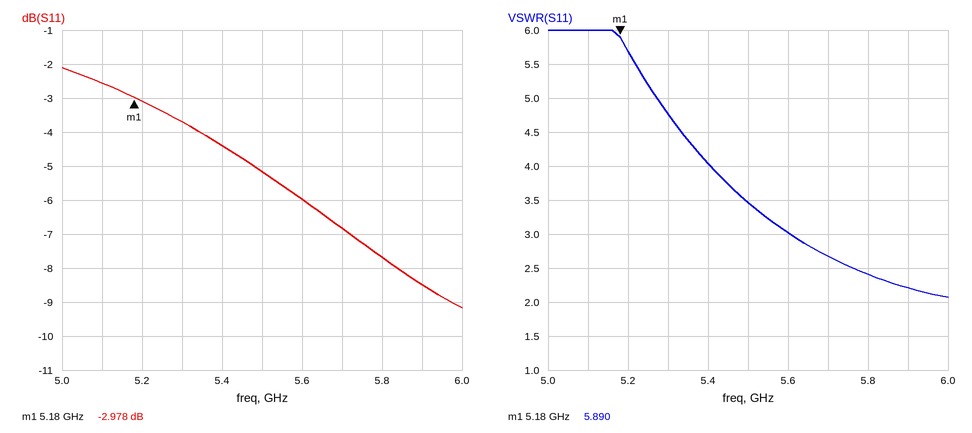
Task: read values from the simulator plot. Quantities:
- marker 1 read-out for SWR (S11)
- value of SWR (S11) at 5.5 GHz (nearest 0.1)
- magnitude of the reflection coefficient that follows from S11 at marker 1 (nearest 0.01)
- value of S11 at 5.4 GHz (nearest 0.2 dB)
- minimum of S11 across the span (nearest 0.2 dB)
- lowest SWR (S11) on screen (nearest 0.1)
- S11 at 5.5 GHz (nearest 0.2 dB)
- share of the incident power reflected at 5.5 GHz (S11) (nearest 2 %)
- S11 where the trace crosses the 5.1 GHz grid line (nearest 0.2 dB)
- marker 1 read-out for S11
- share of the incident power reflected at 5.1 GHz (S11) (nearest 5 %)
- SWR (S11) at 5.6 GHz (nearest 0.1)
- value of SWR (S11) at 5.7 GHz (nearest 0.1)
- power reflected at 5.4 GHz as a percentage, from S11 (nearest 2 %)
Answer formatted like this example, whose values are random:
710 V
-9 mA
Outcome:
5.890
3.5
0.71
-4.4 dB
-9.2 dB
2.1
-5.2 dB
30 %
-2.6 dB
-2.978 dB
55 %
3.0
2.7
36 %
